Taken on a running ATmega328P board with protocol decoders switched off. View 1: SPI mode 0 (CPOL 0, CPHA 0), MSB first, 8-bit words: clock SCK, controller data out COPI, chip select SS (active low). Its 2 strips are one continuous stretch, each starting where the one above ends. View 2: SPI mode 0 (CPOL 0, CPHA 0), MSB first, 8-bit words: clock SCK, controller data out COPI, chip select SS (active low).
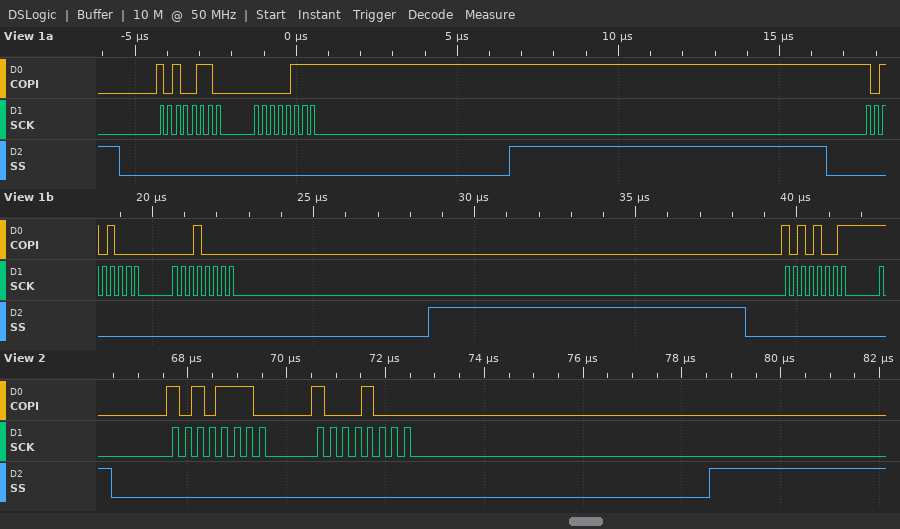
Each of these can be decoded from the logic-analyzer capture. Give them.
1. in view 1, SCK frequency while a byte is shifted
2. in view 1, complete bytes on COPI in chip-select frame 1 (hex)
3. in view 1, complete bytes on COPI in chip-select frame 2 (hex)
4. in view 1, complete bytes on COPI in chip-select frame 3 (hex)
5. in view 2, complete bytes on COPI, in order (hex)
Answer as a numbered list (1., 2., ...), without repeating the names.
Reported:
1. 4 MHz
2. A6 07
3. A8 10
4. A9
5. 0xAE 0x88
